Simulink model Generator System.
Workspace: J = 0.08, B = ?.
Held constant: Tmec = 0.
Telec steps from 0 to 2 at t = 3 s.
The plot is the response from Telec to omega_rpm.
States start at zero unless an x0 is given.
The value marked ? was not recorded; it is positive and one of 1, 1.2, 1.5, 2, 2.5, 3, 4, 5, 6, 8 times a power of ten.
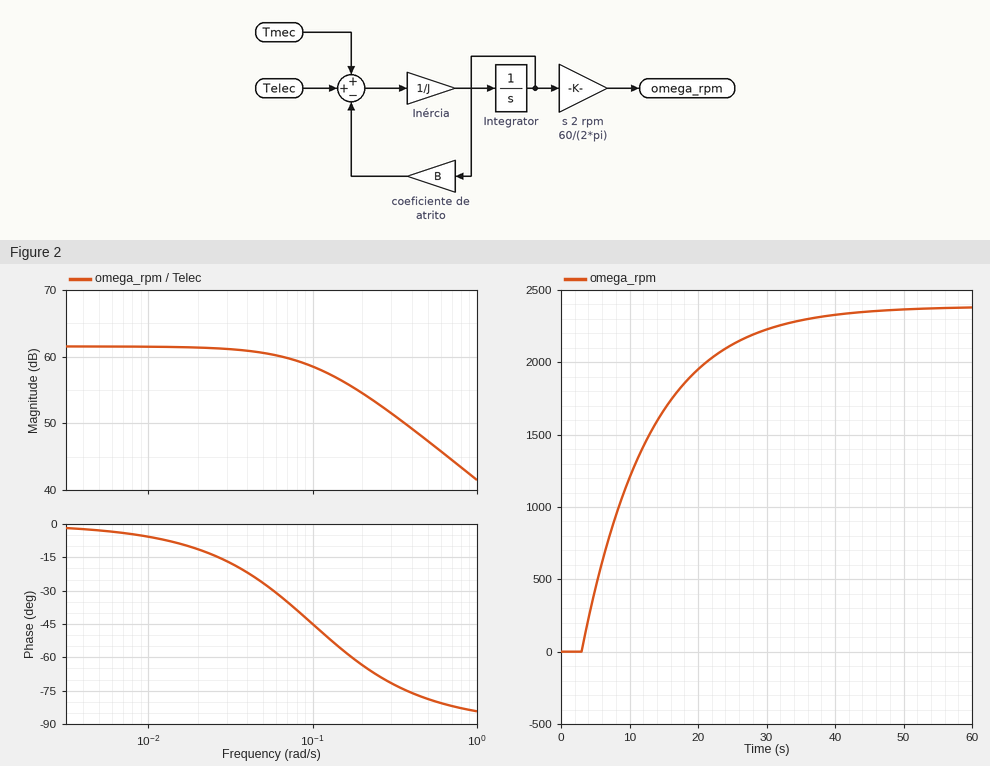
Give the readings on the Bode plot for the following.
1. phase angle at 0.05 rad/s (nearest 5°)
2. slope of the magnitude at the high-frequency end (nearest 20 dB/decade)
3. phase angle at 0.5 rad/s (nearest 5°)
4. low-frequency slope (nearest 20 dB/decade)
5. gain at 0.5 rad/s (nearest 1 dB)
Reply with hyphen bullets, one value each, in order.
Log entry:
- -25°
- -20 dB/decade
- -80°
- 0 dB/decade
- 47 dB
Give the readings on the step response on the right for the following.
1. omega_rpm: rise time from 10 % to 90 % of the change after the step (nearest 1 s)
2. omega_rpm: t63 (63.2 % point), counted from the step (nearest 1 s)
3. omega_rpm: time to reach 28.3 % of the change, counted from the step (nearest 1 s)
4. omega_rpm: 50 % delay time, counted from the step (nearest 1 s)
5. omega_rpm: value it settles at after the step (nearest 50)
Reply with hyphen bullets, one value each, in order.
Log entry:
- 22 s
- 10 s
- 3 s
- 7 s
- 2400
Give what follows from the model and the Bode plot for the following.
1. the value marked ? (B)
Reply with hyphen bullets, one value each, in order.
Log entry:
- 0.008
